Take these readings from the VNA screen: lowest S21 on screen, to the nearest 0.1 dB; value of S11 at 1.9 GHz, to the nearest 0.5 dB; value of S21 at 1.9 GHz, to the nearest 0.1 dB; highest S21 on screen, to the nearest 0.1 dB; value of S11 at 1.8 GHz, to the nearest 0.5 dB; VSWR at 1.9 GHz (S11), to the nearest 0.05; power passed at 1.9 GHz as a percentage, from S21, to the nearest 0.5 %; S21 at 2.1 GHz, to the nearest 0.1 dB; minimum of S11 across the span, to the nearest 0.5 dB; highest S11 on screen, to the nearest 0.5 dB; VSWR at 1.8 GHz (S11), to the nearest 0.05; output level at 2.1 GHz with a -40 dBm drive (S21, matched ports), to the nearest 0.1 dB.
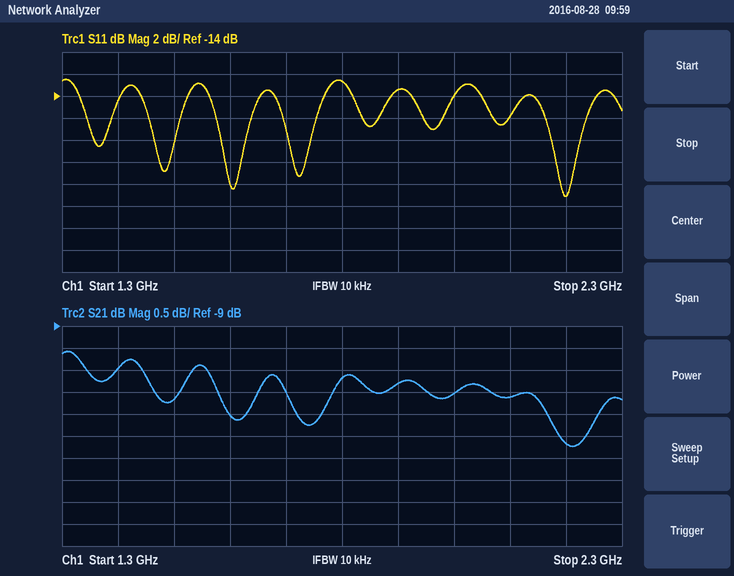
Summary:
-11.7 dB
-13.5 dB
-10.3 dB
-9.6 dB
-12.5 dB
1.55
9.5 %
-10.6 dB
-23.0 dB
-12.5 dB
1.60
-50.6 dBm
